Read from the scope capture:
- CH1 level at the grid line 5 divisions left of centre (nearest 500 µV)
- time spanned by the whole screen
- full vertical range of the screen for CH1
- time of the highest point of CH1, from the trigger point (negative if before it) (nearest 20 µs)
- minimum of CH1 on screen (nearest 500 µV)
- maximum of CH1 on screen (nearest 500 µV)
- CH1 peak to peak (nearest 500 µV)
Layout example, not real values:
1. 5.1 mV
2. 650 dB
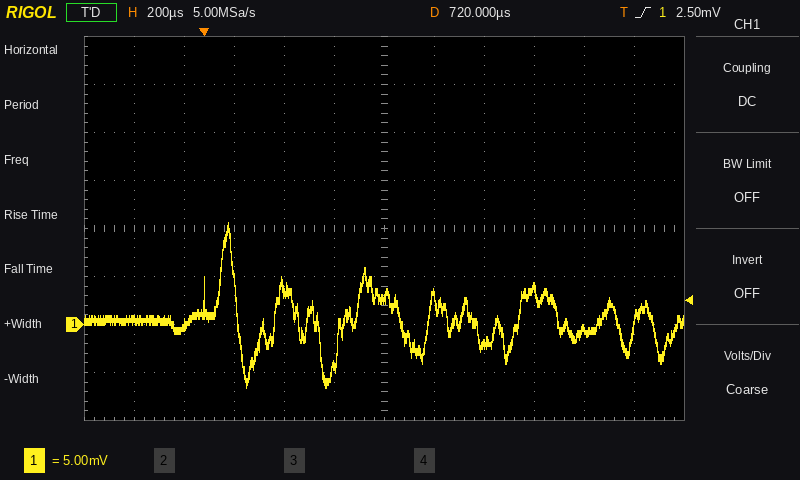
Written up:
1. 500 µV
2. 2.4 ms
3. 40 mV
4. +100 µs
5. -6.5 mV
6. 10.5 mV
7. 17.0 mV
